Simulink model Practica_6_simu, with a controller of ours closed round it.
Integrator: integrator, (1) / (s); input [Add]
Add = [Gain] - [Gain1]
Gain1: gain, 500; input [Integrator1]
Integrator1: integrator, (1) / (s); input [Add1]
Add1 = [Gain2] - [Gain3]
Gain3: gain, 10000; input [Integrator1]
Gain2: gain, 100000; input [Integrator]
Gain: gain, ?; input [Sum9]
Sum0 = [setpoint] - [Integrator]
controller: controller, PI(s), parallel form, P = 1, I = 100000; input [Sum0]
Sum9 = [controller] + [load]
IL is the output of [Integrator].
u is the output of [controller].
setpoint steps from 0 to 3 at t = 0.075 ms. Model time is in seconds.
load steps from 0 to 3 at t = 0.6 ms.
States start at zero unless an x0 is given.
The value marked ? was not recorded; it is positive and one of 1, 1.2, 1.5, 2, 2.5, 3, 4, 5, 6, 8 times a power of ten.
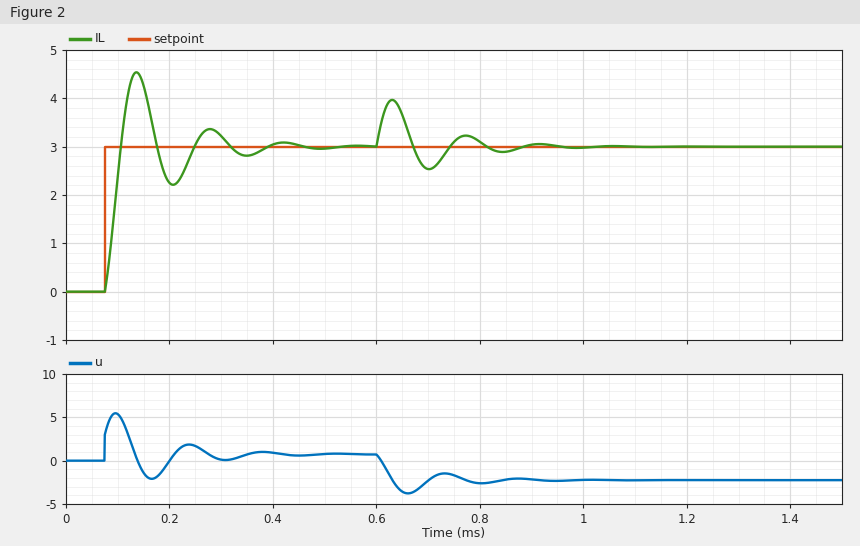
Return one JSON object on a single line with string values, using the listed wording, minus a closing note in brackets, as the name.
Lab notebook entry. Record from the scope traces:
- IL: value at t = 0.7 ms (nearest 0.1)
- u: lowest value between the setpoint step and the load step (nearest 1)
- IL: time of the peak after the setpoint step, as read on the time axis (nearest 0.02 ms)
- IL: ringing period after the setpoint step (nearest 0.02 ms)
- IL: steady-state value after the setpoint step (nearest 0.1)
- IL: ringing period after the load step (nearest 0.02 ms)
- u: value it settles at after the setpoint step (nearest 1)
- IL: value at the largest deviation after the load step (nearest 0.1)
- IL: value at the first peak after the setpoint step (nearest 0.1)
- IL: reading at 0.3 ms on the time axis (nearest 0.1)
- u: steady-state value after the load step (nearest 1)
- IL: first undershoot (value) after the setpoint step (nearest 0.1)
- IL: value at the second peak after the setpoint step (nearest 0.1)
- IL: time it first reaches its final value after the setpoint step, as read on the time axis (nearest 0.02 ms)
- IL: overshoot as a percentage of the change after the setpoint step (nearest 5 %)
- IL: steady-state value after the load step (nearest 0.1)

{"IL: value at t = 0.7 ms": "2.5", "u: lowest value between the setpoint step and the load step": "-2", "IL: time of the peak after the setpoint step, as read on the time axis": "0.14 ms", "IL: ringing period after the setpoint step": "0.14 ms", "IL: steady-state value after the setpoint step": "3.0", "IL: ringing period after the load step": "0.14 ms", "u: value it settles at after the setpoint step": "1", "IL: value at the largest deviation after the load step": "4.0", "IL: value at the first peak after the setpoint step": "4.5", "IL: reading at 0.3 ms on the time axis": "3.2", "u: steady-state value after the load step": "-2", "IL: first undershoot (value) after the setpoint step": "2.2", "IL: value at the second peak after the setpoint step": "3.4", "IL: time it first reaches its final value after the setpoint step, as read on the time axis": "0.10 ms", "IL: overshoot as a percentage of the change after the setpoint step": "50 %", "IL: steady-state value after the load step": "3.0"}
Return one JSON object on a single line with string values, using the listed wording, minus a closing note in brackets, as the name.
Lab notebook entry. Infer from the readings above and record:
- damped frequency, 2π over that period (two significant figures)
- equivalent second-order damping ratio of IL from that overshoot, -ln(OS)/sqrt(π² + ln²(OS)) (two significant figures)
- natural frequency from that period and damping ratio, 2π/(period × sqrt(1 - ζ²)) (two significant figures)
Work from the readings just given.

{"damped frequency, 2π over that period": "45 rad/ms", "equivalent second-order damping ratio of IL from that overshoot, -ln(OS)/sqrt(π² + ln²(OS))": "0.22", "natural frequency from that period and damping ratio, 2π/(period × sqrt(1 - ζ²))": "46 rad/ms"}
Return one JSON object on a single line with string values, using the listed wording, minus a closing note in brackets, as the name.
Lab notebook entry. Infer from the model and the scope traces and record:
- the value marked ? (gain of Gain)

{"the value marked ?": "20000"}
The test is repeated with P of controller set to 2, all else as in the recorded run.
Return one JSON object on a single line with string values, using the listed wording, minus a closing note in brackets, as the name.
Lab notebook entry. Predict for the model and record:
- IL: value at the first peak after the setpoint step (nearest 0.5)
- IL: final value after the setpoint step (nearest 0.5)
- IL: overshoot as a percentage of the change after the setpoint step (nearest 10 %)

{"IL: value at the first peak after the setpoint step": "4.0", "IL: final value after the setpoint step": "3.0", "IL: overshoot as a percentage of the change after the setpoint step": "30 %"}
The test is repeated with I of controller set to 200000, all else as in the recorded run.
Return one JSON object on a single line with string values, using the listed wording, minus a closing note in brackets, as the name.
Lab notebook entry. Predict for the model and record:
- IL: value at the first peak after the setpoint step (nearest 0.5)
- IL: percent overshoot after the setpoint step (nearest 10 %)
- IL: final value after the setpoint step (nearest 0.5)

{"IL: value at the first peak after the setpoint step": "5.0", "IL: percent overshoot after the setpoint step": "60 %", "IL: final value after the setpoint step": "3.0"}
